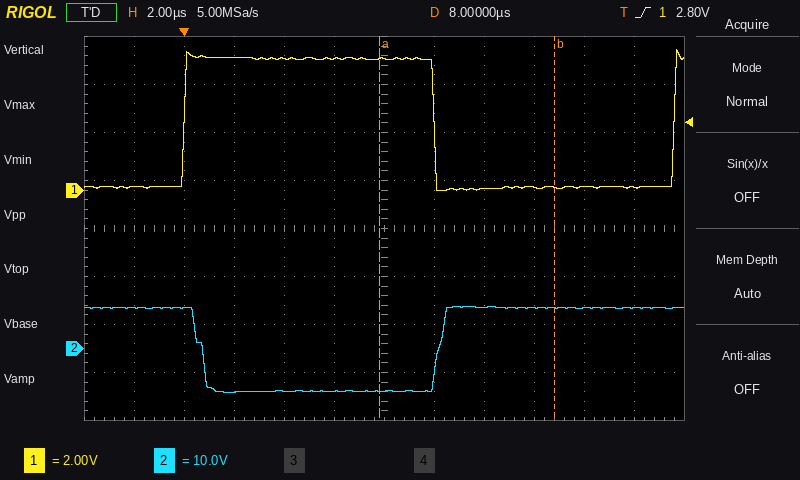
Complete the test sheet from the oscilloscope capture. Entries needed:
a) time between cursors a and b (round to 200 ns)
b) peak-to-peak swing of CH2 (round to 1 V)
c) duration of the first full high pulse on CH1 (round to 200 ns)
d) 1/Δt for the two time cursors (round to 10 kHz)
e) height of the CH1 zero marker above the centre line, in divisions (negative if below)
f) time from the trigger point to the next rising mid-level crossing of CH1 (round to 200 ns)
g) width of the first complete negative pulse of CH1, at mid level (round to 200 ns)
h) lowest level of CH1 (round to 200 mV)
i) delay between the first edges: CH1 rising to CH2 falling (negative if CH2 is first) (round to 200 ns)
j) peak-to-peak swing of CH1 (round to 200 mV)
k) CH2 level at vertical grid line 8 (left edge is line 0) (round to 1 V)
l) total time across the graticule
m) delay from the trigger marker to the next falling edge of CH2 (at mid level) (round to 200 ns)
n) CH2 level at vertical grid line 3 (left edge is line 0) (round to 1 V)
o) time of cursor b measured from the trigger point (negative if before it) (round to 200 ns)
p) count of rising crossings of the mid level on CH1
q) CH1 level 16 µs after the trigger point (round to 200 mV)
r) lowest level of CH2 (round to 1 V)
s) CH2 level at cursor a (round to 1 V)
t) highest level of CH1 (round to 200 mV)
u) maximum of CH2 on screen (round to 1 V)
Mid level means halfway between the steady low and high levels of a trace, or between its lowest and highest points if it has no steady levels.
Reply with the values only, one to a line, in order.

7.0 µs
18 V
10.0 µs
140 kHz
+0.8 div
19.6 µs
9.6 µs
0.0 V
+800 ns
5.8 V
9 V
24 µs
800 ns
-9 V
+14.8 µs
2
200 mV
-9 V
-9 V
5.8 V
9 V
